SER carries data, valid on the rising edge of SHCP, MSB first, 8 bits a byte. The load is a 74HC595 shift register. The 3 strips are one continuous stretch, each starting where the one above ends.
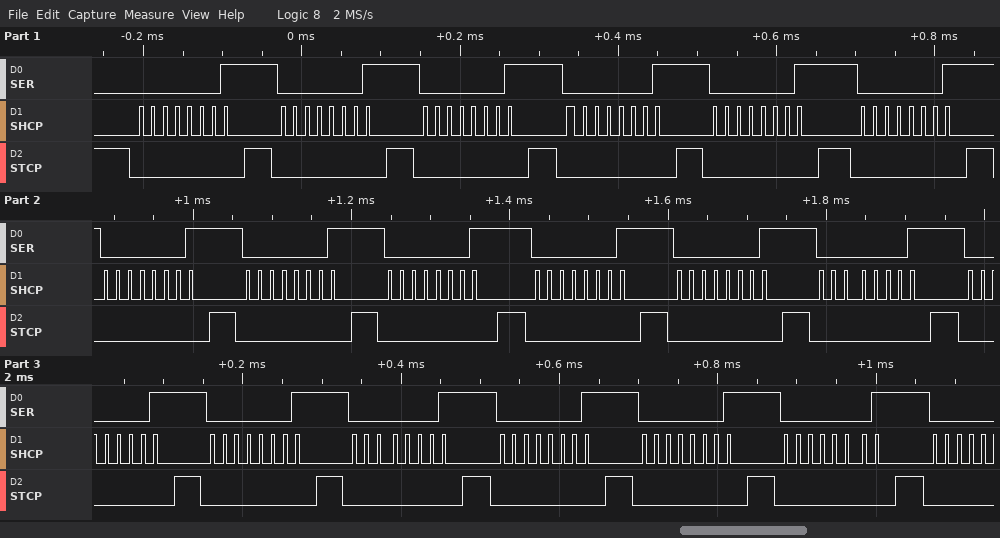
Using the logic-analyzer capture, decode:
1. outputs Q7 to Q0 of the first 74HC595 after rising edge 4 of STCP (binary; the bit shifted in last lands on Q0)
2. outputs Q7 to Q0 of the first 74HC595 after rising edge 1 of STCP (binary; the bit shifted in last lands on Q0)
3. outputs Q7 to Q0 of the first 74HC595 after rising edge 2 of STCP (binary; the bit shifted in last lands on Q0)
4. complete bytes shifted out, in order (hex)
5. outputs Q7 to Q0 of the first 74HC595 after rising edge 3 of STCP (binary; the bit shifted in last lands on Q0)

00000001
00000001
00000001
01 01 01 01 01 01 01 01 01 01 01 01 01 01 01 01 01 01
00000001
